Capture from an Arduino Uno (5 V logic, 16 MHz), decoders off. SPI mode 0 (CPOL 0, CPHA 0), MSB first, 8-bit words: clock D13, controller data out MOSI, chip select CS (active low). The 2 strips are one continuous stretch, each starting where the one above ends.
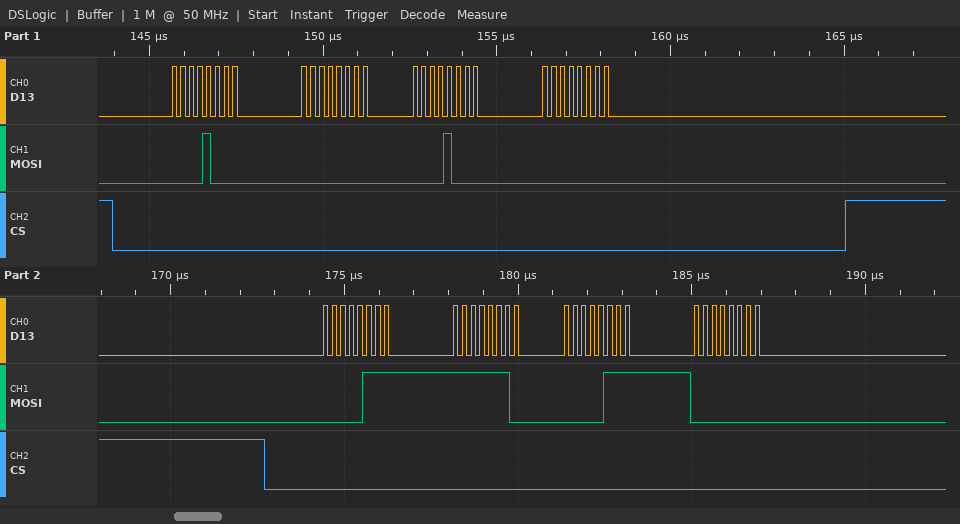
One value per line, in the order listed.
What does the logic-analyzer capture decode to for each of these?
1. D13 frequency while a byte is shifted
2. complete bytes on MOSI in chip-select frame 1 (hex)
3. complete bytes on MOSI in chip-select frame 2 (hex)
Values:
4 MHz
08 00 08 00
07 FE 07 00
